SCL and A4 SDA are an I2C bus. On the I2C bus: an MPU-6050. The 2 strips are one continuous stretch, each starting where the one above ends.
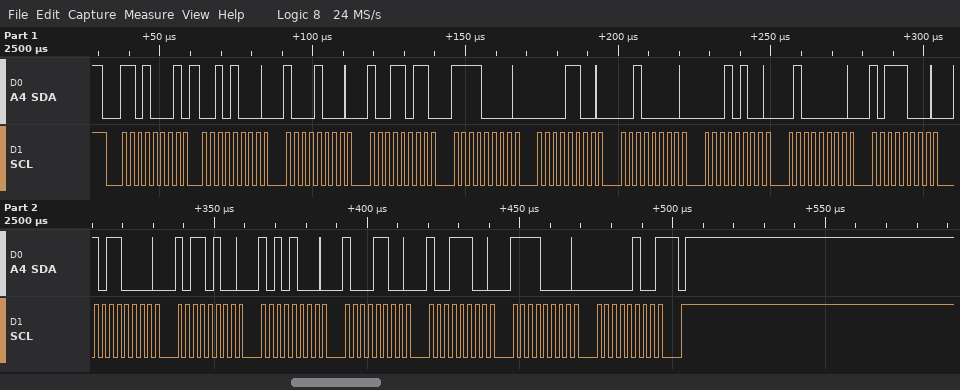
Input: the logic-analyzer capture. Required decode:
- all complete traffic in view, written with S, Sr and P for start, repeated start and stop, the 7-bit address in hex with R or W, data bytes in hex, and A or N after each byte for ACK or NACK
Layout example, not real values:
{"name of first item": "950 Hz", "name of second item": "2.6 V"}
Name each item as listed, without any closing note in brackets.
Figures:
{"all complete traffic in view, written with S, Sr and P for start, repeated start and stop, the 7-bit address in hex with R or W, data bytes in hex, and A or N after each byte for ACK or NACK": "S 68R A 28 A 88 A 9B A F0 A 0C A 20 A 14 A 40 A B8 A B0 A B4 A A8 A 8C A 9C A F0 A 04 N P"}
